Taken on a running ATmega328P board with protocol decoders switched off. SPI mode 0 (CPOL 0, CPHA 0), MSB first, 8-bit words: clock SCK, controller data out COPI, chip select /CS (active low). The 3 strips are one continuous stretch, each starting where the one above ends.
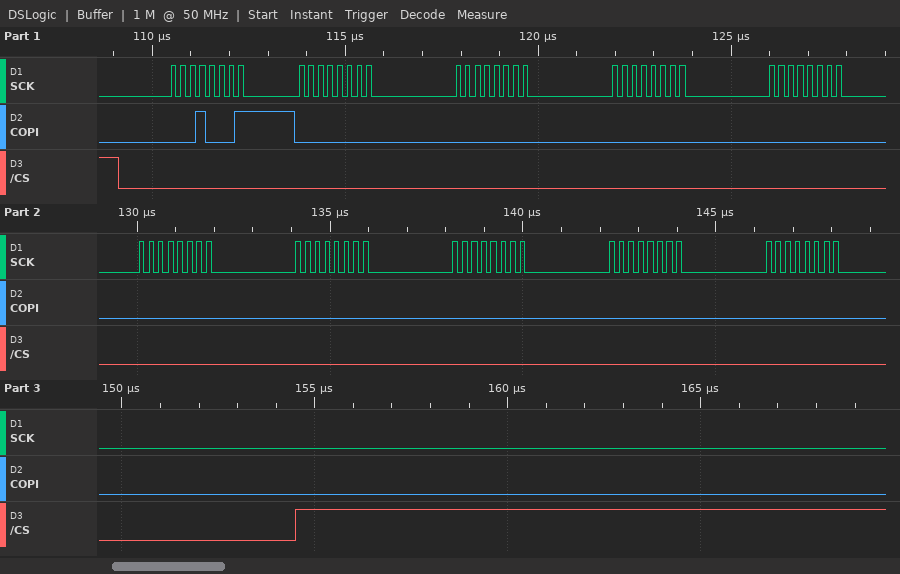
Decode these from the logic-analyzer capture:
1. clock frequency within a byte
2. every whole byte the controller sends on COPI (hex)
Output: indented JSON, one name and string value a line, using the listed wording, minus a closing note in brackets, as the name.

{
  "clock frequency within a byte": "4 MHz",
  "every whole byte the controller sends on COPI": "0x11 0x00 0x00 0x00 0x00 0x00 0x00 0x00 0x00 0x00"
}
